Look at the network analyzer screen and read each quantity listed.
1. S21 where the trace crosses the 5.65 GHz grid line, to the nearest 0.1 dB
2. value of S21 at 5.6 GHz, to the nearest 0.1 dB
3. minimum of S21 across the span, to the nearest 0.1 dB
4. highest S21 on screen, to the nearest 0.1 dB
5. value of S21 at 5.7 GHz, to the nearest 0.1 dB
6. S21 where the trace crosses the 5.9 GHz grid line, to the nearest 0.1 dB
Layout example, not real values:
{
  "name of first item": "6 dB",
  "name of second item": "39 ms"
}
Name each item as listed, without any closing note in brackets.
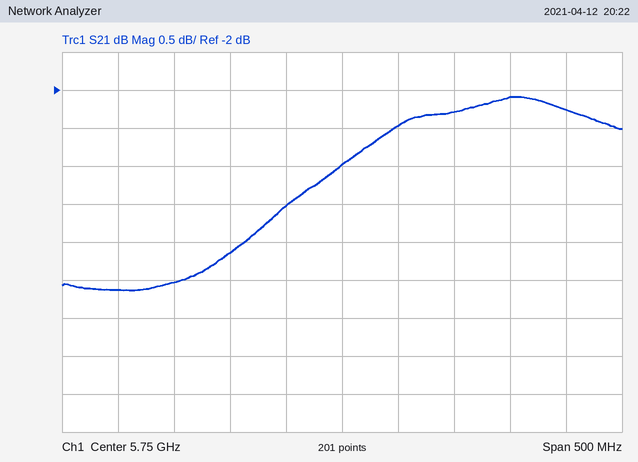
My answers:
{
  "S21 where the trace crosses the 5.65 GHz grid line, to the nearest 0.1 dB": "-4.1 dB",
  "value of S21 at 5.6 GHz, to the nearest 0.1 dB": "-4.5 dB",
  "minimum of S21 across the span, to the nearest 0.1 dB": "-4.6 dB",
  "highest S21 on screen, to the nearest 0.1 dB": "-2.1 dB",
  "value of S21 at 5.7 GHz, to the nearest 0.1 dB": "-3.5 dB",
  "S21 where the trace crosses the 5.9 GHz grid line, to the nearest 0.1 dB": "-2.1 dB"
}
